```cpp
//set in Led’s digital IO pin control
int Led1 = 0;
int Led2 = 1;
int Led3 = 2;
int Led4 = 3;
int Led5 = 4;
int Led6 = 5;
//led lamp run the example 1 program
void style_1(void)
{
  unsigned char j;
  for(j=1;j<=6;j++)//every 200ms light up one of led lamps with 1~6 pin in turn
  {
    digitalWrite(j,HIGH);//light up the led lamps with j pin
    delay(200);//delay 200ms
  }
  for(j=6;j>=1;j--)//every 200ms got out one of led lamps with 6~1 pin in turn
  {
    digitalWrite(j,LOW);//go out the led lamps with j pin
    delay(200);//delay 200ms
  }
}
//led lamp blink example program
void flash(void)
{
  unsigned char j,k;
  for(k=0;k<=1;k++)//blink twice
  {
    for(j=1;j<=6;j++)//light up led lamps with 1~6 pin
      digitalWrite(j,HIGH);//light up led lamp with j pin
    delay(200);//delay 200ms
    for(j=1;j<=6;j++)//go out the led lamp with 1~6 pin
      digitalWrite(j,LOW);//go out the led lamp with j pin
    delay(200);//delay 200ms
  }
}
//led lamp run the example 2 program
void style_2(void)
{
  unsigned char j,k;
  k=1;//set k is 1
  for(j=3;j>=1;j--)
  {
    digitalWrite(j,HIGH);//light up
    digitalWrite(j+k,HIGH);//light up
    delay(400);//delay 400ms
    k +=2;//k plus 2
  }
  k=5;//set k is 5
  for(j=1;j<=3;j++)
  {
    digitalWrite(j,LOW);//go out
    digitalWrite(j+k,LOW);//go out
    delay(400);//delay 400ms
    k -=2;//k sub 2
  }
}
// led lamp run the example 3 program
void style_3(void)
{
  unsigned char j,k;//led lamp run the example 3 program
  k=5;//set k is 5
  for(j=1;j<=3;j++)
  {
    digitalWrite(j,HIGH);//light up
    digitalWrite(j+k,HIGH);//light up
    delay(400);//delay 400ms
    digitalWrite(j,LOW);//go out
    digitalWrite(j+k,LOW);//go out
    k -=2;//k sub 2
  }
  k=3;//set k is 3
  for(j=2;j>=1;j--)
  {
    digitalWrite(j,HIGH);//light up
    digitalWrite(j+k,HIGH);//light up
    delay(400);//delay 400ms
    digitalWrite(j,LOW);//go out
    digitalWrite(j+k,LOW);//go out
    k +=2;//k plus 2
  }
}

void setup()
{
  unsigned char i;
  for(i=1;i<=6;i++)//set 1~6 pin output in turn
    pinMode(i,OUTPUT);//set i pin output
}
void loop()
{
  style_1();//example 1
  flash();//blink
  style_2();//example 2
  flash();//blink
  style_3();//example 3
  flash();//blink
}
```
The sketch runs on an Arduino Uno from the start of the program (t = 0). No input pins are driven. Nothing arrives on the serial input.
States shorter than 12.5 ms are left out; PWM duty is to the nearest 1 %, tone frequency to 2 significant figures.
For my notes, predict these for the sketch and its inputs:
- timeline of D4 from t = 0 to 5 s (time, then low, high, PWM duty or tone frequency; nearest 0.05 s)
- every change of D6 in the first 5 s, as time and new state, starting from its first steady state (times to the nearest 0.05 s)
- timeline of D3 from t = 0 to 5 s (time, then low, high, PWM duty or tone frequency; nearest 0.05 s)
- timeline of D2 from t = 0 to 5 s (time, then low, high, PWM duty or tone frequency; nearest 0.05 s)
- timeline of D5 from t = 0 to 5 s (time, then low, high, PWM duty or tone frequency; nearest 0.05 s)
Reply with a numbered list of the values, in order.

1. 0 s low; 0.6 s high; 1.6 s low; 2.4 s high; 2.6 s low; 2.8 s high; 3 s low; 3.2 s high
2. 0 s low; 1 s high; 1.2 s low; 2.4 s high; 2.6 s low; 2.8 s high; 3 s low; 4 s high; 4.4 s low
3. 0 s low; 0.4 s high; 1.8 s low; 2.4 s high; 2.6 s low; 2.8 s high; 3 s low; 3.2 s high
4. 0 s low; 0.2 s high; 2 s low; 2.4 s high; 2.6 s low; 2.8 s high; 3 s low; 3.6 s high; 4.8 s low
5. 0 s low; 0.8 s high; 1.4 s low; 2.4 s high; 2.6 s low; 2.8 s high; 3 s low; 3.6 s high; 4.8 s low
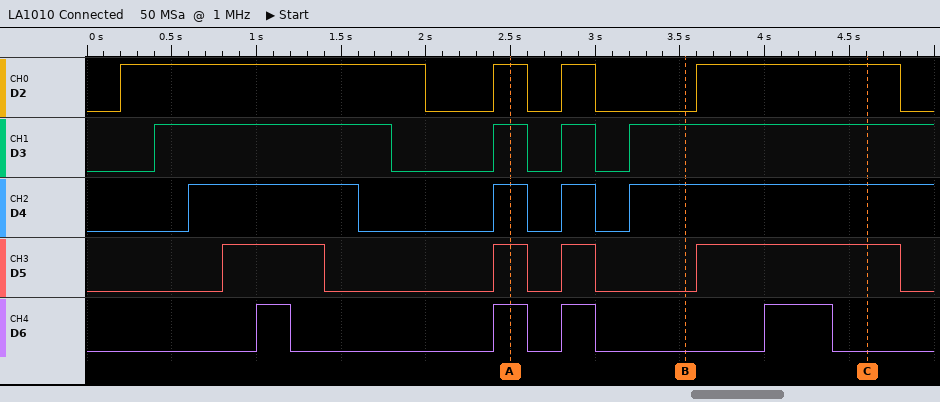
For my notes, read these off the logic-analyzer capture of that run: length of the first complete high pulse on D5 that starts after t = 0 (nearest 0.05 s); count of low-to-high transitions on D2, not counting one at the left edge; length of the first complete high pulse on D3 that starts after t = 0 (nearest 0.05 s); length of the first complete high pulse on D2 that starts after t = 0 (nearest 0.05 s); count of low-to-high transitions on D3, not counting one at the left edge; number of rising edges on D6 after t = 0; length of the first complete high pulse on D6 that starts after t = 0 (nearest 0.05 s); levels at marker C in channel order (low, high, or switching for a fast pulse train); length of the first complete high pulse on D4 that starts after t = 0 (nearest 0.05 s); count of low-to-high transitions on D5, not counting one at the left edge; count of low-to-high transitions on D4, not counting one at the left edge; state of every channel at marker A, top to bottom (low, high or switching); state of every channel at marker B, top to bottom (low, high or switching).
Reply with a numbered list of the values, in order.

1. 0.60 s
2. 4
3. 1.40 s
4. 1.80 s
5. 4
6. 4
7. 0.20 s
8. D2 high, D3 high, D4 high, D5 high, D6 low
9. 1.00 s
10. 4
11. 4
12. D2 high, D3 high, D4 high, D5 high, D6 high
13. D2 low, D3 high, D4 high, D5 low, D6 low
